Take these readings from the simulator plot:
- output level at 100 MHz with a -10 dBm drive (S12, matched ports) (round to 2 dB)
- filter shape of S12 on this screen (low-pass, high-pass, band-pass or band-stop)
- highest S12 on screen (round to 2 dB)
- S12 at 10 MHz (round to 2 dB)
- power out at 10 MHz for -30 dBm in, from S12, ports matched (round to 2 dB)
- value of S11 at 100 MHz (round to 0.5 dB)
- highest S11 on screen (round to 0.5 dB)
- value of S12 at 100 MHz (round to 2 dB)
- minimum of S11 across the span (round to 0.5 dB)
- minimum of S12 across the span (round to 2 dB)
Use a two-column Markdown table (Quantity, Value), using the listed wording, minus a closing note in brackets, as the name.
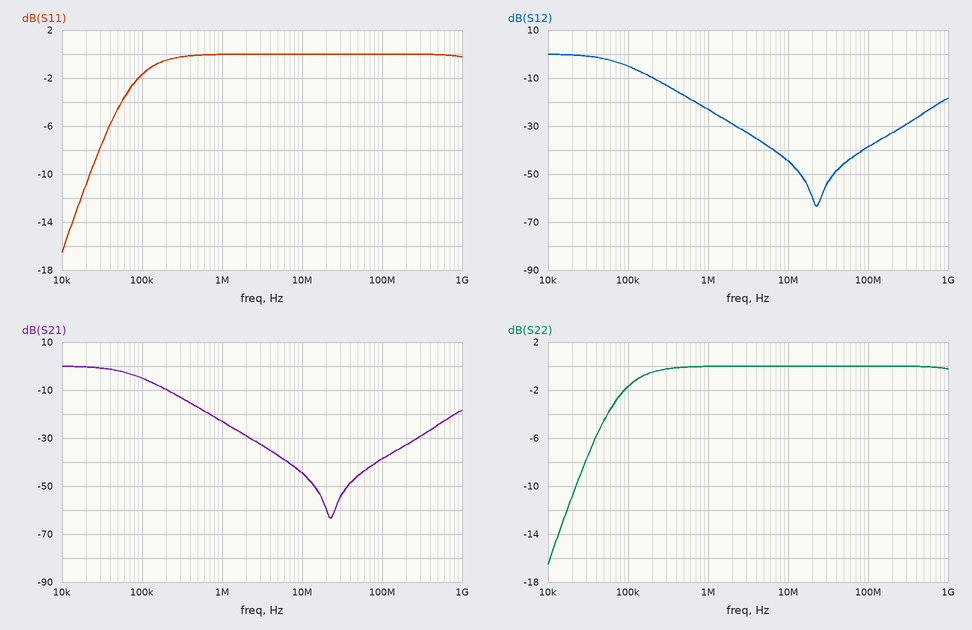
| Quantity | Value |
|---|---|
| output level at 100 MHz with a -10 dBm drive (S12, matched ports) | -48 dBm |
| filter shape of S12 on this screen | low-pass |
| highest S12 on screen | 0 dB |
| S12 at 10 MHz | -44 dB |
| power out at 10 MHz for -30 dBm in, from S12, ports matched | -74 dBm |
| value of S11 at 100 MHz | 0.0 dB |
| highest S11 on screen | 0.0 dB |
| value of S12 at 100 MHz | -38 dB |
| minimum of S11 across the span | -16.5 dB |
| minimum of S12 across the span | -64 dB |
